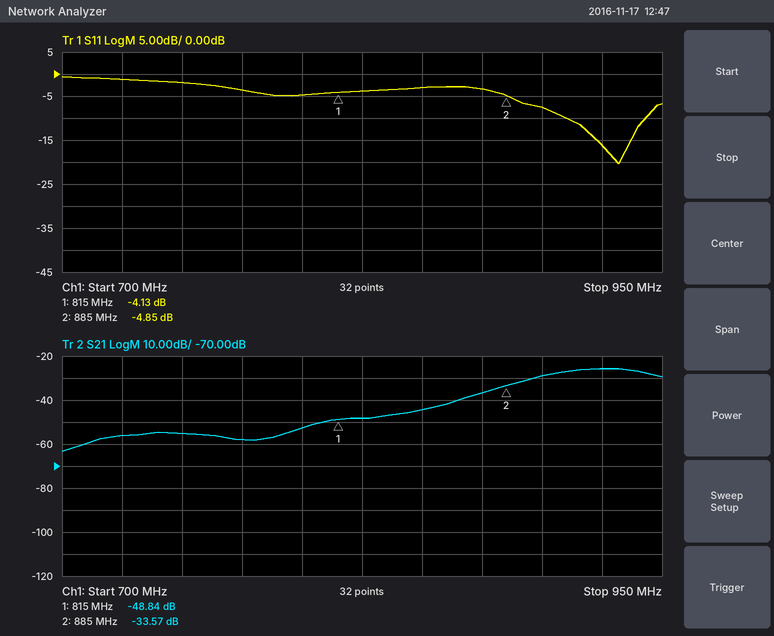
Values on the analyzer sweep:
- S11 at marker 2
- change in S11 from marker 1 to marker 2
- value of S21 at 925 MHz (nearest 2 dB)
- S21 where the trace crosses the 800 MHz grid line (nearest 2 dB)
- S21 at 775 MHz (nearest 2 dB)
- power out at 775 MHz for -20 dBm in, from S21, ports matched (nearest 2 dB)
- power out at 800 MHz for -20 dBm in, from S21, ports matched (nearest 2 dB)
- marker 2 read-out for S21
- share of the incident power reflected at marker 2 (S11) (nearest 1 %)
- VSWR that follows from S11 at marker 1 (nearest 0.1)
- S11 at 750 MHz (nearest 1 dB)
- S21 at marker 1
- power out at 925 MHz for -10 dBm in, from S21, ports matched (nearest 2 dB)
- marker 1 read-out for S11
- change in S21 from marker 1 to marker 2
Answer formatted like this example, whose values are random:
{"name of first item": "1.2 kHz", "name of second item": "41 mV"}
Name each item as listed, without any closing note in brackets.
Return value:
{"S11 at marker 2": "-4.85 dB", "change in S11 from marker 1 to marker 2": "-0.72 dB", "value of S21 at 925 MHz": "-26 dB", "S21 where the trace crosses the 800 MHz grid line": "-52 dB", "S21 at 775 MHz": "-58 dB", "power out at 775 MHz for -20 dBm in, from S21, ports matched": "-78 dBm", "power out at 800 MHz for -20 dBm in, from S21, ports matched": "-72 dBm", "marker 2 read-out for S21": "-33.57 dB", "share of the incident power reflected at marker 2 (S11)": "33 %", "VSWR that follows from S11 at marker 1": "4.3", "S11 at 750 MHz": "-2 dB", "S21 at marker 1": "-48.84 dB", "power out at 925 MHz for -10 dBm in, from S21, ports matched": "-36 dBm", "marker 1 read-out for S11": "-4.13 dB", "change in S21 from marker 1 to marker 2": "15.27 dB"}
